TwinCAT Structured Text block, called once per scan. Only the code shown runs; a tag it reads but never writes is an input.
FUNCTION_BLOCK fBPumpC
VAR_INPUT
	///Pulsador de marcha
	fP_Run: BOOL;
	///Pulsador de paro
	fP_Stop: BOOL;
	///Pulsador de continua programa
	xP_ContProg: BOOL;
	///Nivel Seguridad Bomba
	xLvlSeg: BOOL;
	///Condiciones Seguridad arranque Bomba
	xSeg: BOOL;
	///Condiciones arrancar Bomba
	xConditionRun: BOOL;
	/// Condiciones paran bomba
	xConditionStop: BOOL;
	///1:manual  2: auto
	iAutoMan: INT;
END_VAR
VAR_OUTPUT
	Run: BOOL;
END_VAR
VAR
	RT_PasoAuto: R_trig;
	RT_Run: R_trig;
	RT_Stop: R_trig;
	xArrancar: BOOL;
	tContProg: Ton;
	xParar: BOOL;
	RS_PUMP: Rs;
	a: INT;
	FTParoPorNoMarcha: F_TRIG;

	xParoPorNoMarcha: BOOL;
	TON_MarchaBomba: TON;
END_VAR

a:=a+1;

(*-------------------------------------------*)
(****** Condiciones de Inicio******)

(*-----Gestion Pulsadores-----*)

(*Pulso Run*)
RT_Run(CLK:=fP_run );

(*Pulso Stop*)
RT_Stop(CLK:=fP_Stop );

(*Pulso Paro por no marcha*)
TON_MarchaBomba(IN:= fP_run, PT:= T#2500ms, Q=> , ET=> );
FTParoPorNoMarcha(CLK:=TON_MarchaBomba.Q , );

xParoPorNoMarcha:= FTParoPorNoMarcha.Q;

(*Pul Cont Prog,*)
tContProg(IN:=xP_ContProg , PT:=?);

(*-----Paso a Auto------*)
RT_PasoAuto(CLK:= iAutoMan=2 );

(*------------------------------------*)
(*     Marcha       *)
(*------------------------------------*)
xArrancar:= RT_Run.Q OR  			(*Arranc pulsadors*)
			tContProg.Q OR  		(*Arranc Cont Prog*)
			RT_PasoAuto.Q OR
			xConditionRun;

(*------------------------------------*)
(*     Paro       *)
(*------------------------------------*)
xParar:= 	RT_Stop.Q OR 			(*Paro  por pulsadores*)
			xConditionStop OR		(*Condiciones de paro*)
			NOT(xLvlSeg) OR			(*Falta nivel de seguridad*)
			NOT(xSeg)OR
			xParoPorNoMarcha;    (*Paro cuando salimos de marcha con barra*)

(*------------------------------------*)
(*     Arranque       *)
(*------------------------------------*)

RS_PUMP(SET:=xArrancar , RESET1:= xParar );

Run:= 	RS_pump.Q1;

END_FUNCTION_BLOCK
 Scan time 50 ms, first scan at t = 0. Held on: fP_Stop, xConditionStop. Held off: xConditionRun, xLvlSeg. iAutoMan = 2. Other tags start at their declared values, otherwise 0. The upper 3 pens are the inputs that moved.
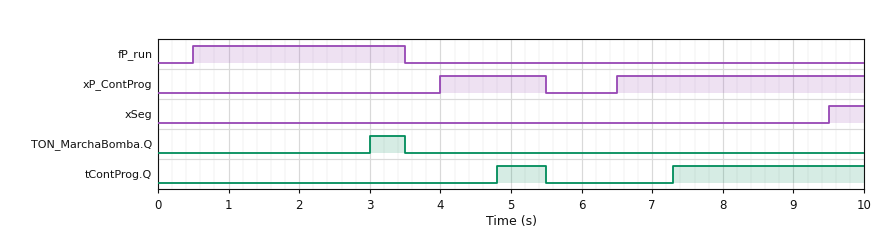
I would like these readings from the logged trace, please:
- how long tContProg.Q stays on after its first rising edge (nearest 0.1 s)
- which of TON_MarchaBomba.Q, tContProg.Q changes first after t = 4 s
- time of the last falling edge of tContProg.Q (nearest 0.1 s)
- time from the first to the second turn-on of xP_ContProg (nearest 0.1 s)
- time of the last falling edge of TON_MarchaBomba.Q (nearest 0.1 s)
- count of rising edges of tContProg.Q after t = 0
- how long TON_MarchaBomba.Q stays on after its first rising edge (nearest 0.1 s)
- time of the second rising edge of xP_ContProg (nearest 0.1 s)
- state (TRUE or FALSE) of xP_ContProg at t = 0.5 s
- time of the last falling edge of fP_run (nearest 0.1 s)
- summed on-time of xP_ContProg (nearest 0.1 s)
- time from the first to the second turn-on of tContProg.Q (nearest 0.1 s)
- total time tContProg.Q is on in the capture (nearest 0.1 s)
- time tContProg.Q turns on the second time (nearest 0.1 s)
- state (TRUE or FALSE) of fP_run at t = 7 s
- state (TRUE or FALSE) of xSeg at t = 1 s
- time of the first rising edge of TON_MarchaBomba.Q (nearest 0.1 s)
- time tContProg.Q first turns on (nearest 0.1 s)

0.7 s
tContProg.Q
5.5 s
2.5 s
3.5 s
2
0.5 s
6.5 s
FALSE
3.5 s
5.0 s
2.5 s
3.4 s
7.3 s
FALSE
FALSE
3.0 s
4.8 s
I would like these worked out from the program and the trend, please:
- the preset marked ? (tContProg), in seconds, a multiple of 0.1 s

0.8 s
